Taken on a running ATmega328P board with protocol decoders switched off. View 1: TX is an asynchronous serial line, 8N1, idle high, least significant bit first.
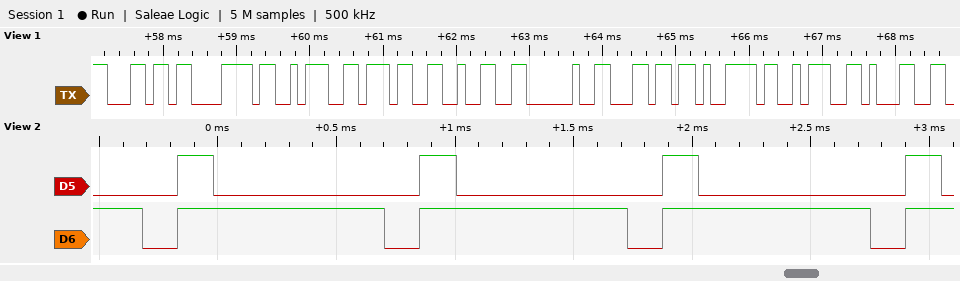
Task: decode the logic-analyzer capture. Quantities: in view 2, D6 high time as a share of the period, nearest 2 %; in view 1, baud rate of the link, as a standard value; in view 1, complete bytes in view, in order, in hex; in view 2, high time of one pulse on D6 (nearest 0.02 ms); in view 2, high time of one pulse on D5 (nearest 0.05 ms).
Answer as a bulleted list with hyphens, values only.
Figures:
- 86 %
- 9600 baud
- 6C 78 3A 37 32 20 6C 79 3A 31
- 0.88 ms
- 0.15 ms
